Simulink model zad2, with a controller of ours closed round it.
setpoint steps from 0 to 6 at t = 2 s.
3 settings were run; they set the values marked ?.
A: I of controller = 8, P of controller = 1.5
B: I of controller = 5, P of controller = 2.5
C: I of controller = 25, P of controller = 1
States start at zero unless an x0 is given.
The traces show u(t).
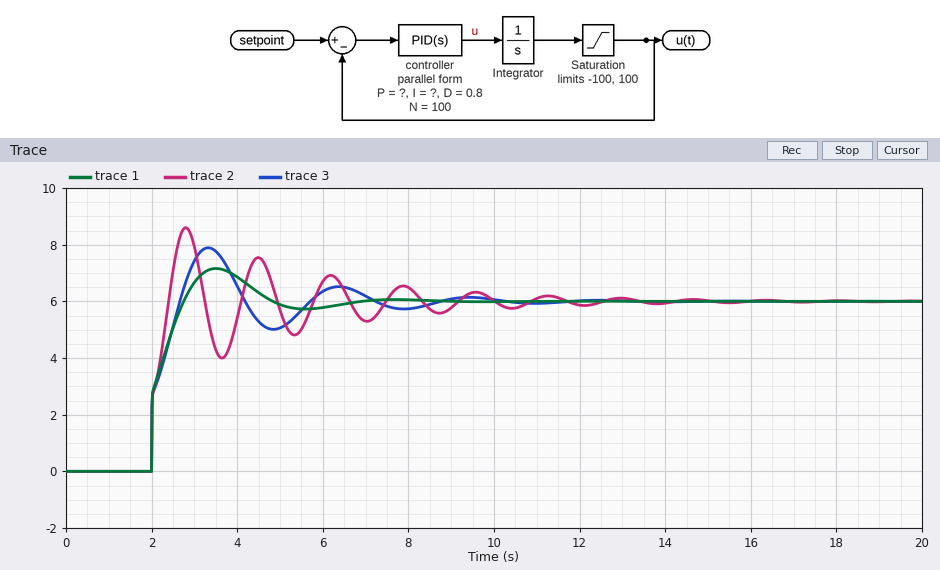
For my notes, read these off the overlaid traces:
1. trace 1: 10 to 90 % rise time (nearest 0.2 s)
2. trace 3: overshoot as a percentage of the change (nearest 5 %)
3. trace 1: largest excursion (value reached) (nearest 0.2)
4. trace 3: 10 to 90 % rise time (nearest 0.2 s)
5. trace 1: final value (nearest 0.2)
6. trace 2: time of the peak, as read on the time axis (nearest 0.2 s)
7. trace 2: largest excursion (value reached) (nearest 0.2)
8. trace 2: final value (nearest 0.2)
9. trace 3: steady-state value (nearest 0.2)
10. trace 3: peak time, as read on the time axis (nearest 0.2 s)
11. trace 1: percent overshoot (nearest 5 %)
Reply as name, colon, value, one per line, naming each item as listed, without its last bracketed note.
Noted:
trace 1: 10 to 90 % rise time: 0.6 s
trace 3: overshoot as a percentage of the change: 30 %
trace 1: largest excursion (value reached): 7.2
trace 3: 10 to 90 % rise time: 0.6 s
trace 1: final value: 6.0
trace 2: time of the peak, as read on the time axis: 2.8 s
trace 2: largest excursion (value reached): 8.6
trace 2: final value: 6.0
trace 3: steady-state value: 6.0
trace 3: peak time, as read on the time axis: 3.4 s
trace 1: percent overshoot: 20 %
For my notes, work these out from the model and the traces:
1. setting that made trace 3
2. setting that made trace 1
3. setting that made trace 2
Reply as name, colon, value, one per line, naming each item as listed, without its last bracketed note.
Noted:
setting that made trace 3: A
setting that made trace 1: B
setting that made trace 2: C
